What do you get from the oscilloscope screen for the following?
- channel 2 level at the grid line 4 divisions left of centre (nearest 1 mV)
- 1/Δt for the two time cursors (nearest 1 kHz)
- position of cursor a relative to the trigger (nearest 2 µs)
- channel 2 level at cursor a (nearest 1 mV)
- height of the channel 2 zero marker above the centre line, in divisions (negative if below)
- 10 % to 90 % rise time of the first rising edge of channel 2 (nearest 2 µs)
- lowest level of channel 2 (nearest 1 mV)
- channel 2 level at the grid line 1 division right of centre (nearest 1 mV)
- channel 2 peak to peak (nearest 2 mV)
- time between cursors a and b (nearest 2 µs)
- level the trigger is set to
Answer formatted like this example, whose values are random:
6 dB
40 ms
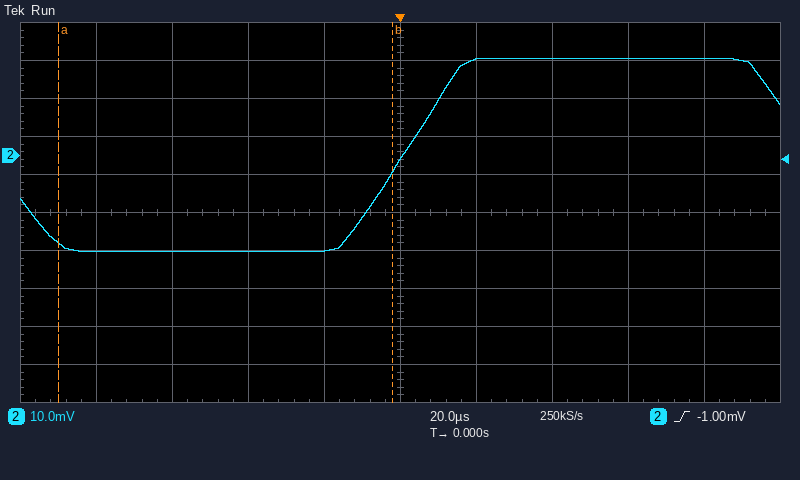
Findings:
-25 mV
11 kHz
-90 µs
-23 mV
+1.5 div
26 µs
-25 mV
25 mV
50 mV
88 µs
-1.00 mV
